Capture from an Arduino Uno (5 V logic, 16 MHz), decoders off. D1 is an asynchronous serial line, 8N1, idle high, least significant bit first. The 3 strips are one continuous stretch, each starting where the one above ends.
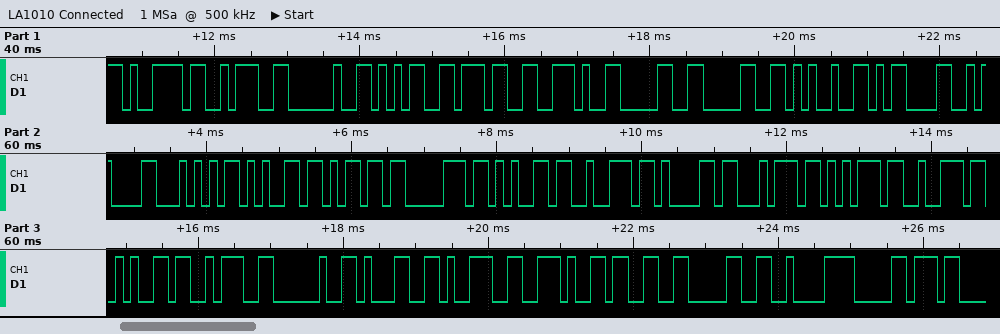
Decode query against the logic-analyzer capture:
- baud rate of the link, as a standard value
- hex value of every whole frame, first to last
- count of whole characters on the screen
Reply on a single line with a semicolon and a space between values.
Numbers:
9600 baud; 79 3A 20 35 37 2E 30 30 25 0D 0A 54 65 6D 70 65 72 61 74 75 72 65 3A 20 31 39 2E 33 30 C2 B0; 31
